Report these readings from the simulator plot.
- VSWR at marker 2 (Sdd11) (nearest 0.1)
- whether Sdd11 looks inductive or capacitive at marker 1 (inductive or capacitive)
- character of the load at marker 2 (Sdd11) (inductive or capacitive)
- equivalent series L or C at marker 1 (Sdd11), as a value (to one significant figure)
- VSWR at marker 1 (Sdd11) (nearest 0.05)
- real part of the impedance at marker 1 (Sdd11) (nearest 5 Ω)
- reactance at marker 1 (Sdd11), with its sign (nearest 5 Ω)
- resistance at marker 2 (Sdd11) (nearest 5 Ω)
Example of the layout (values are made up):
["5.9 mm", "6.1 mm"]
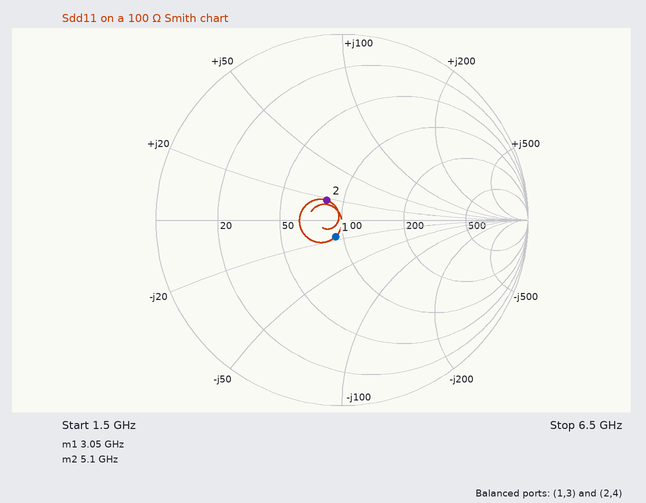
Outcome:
["1.3", "capacitive", "inductive", "3 pF", "1.20", "90 Ω", "-15 Ω", "85 Ω"]
